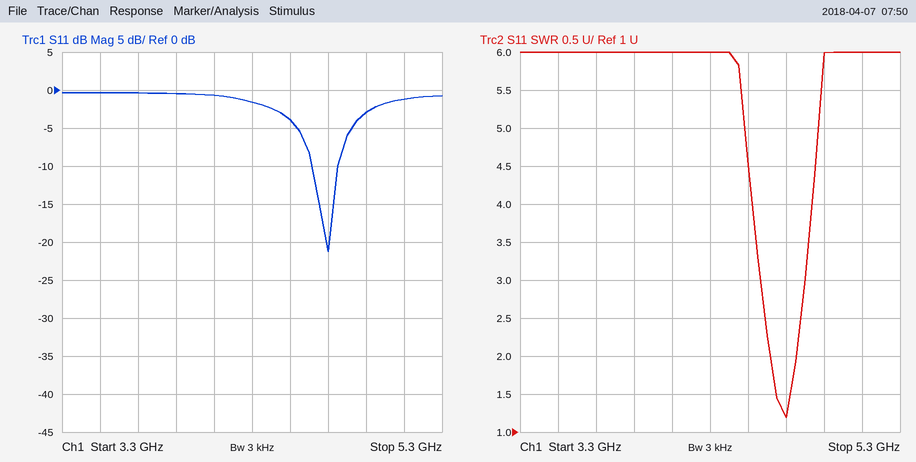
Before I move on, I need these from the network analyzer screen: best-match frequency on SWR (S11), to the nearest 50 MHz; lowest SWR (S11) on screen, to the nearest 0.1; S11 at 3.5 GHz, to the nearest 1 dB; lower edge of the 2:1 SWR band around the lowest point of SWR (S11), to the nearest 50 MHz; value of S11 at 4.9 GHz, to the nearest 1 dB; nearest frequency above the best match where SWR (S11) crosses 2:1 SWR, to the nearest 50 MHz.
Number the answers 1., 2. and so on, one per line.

1. 4.70 GHz
2. 1.2
3. 0 dB
4. 4.60 GHz
5. -3 dB
6. 4.75 GHz
